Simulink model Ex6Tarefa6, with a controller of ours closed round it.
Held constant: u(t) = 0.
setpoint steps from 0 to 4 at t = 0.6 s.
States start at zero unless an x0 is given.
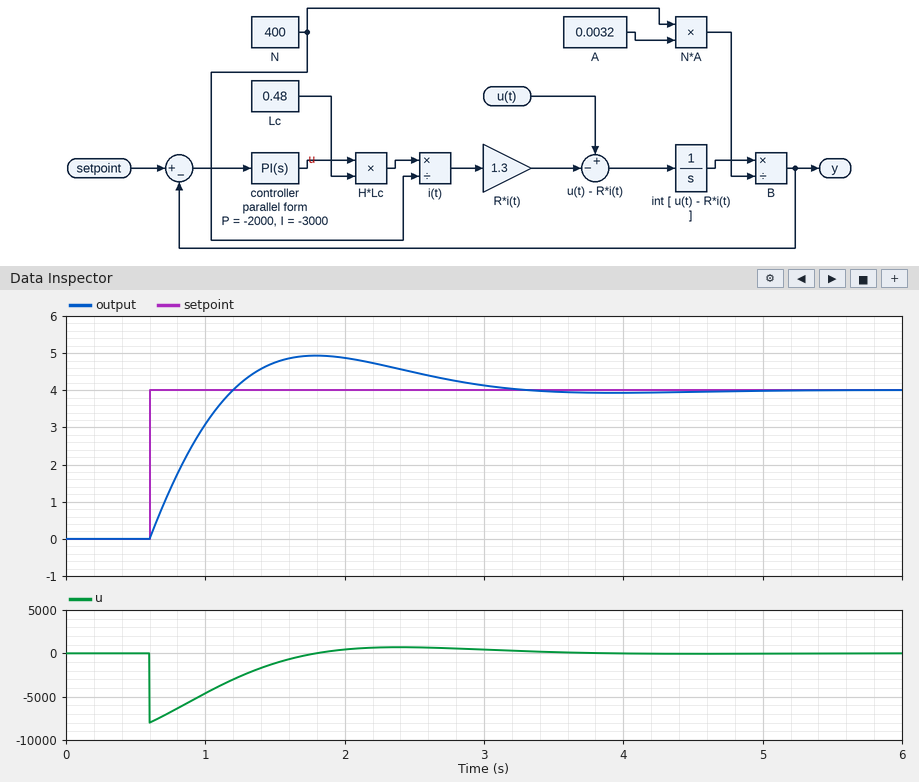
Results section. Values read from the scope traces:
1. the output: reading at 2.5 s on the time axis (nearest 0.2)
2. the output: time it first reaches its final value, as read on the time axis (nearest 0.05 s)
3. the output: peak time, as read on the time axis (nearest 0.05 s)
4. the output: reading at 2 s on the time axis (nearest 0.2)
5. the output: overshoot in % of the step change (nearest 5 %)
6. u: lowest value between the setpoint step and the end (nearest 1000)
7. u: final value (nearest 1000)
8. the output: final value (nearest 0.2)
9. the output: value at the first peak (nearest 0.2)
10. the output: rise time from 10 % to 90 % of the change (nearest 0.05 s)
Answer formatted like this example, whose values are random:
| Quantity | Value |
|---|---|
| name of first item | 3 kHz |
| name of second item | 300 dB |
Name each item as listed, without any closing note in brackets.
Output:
| Quantity | Value |
|---|---|
| the output: reading at 2.5 s on the time axis | 4.4 |
| the output: time it first reaches its final value, as read on the time axis | 1.20 s |
| the output: peak time, as read on the time axis | 1.80 s |
| the output: reading at 2 s on the time axis | 4.8 |
| the output: overshoot in % of the step change | 25 % |
| u: lowest value between the setpoint step and the end | -8000 |
| u: final value | 0 |
| the output: final value | 4.0 |
| the output: value at the first peak | 5.0 |
| the output: rise time from 10 % to 90 % of the change | 0.45 s |
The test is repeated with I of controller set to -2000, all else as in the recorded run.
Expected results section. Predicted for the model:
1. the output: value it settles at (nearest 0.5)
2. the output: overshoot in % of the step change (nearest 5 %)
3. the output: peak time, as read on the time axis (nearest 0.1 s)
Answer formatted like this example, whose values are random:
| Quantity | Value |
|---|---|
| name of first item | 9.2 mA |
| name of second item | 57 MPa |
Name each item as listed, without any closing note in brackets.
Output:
| Quantity | Value |
|---|---|
| the output: value it settles at | 4.0 |
| the output: overshoot in % of the step change | 20 % |
| the output: peak time, as read on the time axis | 2.0 s |
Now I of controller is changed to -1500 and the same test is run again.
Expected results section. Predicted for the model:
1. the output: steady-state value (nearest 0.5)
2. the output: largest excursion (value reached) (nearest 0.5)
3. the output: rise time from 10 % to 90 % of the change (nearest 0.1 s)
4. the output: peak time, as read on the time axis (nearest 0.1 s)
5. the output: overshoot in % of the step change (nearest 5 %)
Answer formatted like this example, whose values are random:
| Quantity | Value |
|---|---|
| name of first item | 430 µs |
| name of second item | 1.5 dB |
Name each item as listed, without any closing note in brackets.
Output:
| Quantity | Value |
|---|---|
| the output: steady-state value | 4.0 |
| the output: largest excursion (value reached) | 4.5 |
| the output: rise time from 10 % to 90 % of the change | 0.6 s |
| the output: peak time, as read on the time axis | 2.1 s |
| the output: overshoot in % of the step change | 15 % |
